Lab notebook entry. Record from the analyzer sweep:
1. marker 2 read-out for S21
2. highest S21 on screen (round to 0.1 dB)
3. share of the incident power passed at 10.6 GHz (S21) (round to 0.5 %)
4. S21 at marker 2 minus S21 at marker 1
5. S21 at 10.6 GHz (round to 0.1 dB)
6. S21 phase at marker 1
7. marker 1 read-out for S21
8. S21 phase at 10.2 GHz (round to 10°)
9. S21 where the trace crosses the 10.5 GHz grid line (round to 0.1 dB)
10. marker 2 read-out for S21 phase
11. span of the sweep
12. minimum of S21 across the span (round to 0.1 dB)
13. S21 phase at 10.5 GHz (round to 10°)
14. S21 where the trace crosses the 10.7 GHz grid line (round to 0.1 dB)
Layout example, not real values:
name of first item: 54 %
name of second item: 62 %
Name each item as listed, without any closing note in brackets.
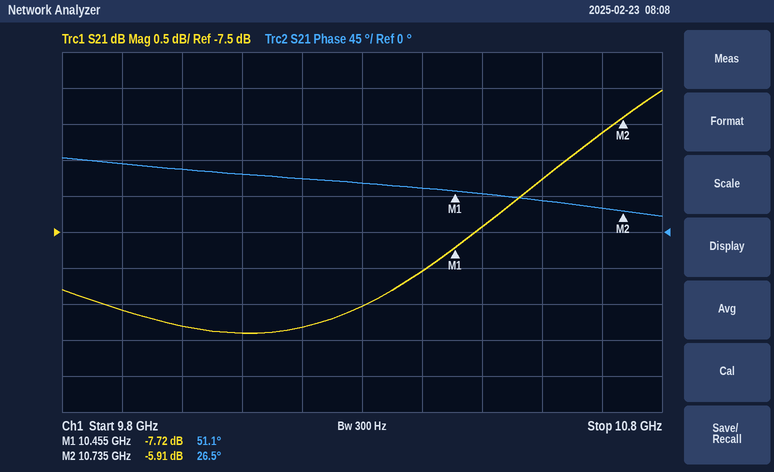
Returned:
marker 2 read-out for S21: -5.91 dB
highest S21 on screen: -5.5 dB
share of the incident power passed at 10.6 GHz (S21): 21.0 %
S21 at marker 2 minus S21 at marker 1: 1.81 dB
S21 at 10.6 GHz: -6.8 dB
S21 phase at marker 1: 51.1°
marker 1 read-out for S21: -7.72 dB
S21 phase at 10.2 GHz: 70°
S21 where the trace crosses the 10.5 GHz grid line: -7.4 dB
marker 2 read-out for S21 phase: 26.5°
span of the sweep: 1 GHz
minimum of S21 across the span: -8.9 dB
S21 phase at 10.5 GHz: 50°
S21 where the trace crosses the 10.7 GHz grid line: -6.1 dB
